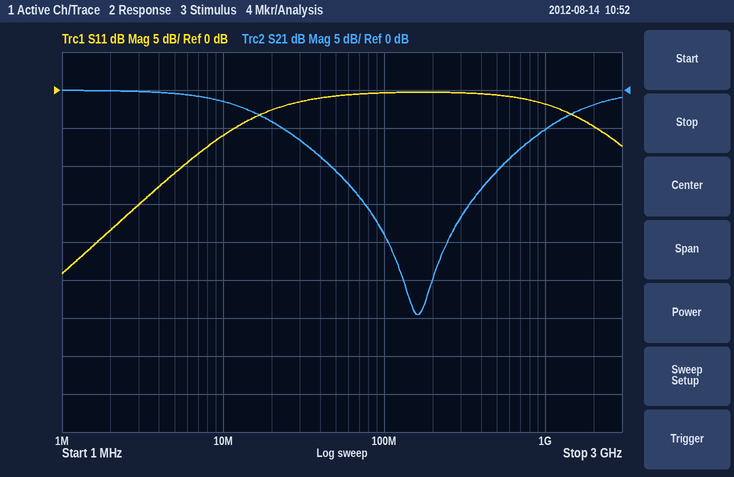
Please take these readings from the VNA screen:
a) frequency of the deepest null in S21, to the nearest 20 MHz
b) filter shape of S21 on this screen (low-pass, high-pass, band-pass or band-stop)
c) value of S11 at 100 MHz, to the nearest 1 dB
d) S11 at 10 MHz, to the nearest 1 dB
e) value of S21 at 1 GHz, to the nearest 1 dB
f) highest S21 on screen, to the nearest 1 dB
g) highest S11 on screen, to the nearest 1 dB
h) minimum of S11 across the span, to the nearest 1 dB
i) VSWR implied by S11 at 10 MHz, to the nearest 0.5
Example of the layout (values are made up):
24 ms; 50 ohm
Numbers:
160 MHz; band-stop; 0 dB; -6 dB; -5 dB; 0 dB; 0 dB; -24 dB; 3.0
